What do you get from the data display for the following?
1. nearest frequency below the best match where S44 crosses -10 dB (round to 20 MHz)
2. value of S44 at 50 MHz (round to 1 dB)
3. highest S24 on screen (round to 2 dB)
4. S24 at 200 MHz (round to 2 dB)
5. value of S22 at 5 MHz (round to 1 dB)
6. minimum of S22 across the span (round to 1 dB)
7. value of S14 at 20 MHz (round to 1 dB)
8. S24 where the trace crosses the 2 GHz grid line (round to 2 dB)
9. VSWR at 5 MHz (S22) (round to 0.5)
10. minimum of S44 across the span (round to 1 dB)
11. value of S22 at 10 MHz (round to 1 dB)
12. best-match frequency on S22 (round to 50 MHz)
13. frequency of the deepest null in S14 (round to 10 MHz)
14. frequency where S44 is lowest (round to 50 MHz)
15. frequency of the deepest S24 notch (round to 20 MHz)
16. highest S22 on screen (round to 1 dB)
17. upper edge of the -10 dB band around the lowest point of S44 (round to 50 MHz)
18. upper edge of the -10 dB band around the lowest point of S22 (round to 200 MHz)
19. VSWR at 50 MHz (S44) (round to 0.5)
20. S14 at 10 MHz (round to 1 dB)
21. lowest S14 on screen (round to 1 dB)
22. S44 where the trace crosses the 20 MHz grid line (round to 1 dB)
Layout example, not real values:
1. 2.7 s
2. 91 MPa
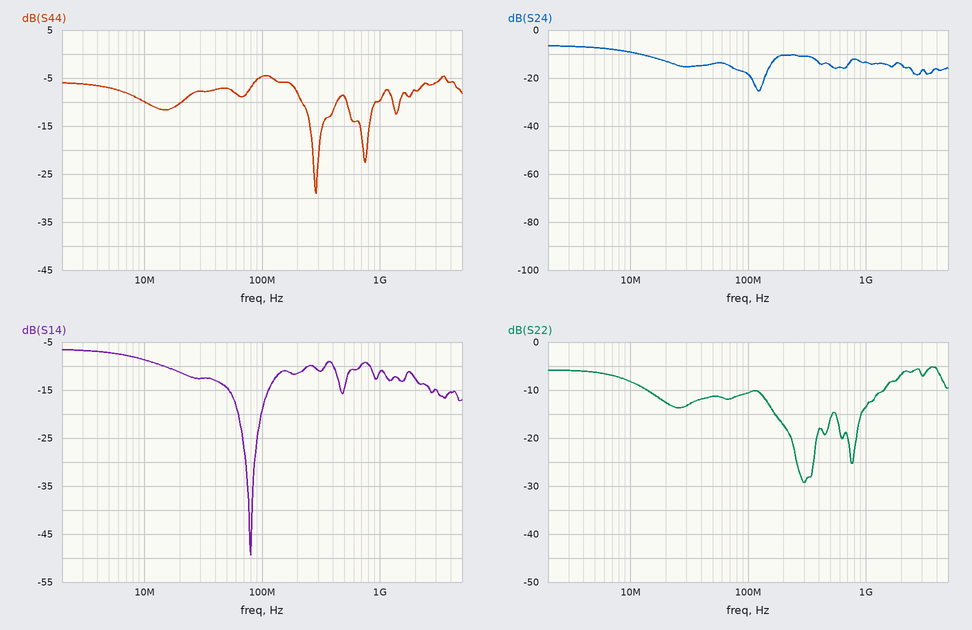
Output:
1. 220 MHz
2. -7 dB
3. -6 dB
4. -10 dB
5. -6 dB
6. -29 dB
7. -11 dB
8. -14 dB
9. 3.0
10. -29 dB
11. -8 dB
12. 300 MHz
13. 80 MHz
14. 300 MHz
15. 120 MHz
16. -5 dB
17. 450 MHz
18. 1.4 GHz
19. 2.5
20. -9 dB
21. -49 dB
22. -10 dB
